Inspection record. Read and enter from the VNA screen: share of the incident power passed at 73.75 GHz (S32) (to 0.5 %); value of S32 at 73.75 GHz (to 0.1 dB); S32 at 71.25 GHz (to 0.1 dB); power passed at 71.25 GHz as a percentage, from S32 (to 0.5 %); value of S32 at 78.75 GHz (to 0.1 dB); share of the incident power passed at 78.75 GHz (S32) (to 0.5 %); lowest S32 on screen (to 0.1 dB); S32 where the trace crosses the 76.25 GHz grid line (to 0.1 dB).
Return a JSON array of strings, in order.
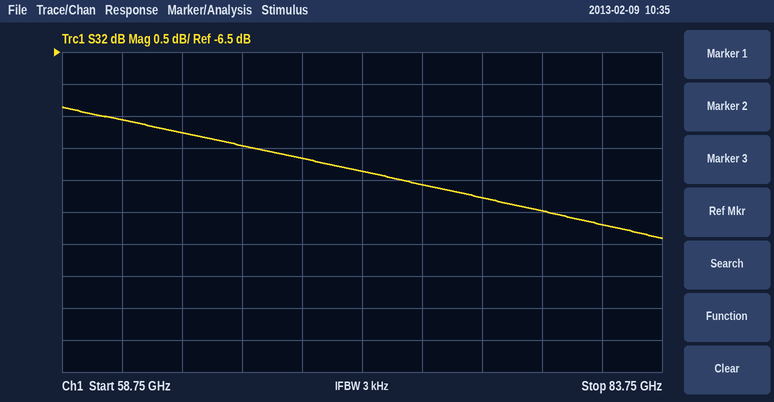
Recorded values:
["14.0 %", "-8.6 dB", "-8.4 dB", "14.5 %", "-9.0 dB", "12.5 %", "-9.4 dB", "-8.8 dB"]
